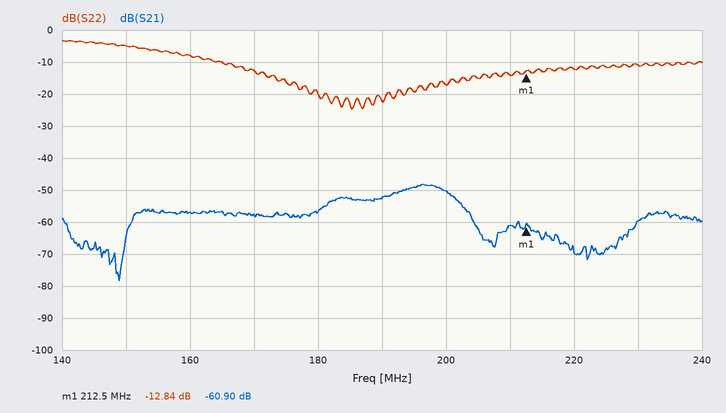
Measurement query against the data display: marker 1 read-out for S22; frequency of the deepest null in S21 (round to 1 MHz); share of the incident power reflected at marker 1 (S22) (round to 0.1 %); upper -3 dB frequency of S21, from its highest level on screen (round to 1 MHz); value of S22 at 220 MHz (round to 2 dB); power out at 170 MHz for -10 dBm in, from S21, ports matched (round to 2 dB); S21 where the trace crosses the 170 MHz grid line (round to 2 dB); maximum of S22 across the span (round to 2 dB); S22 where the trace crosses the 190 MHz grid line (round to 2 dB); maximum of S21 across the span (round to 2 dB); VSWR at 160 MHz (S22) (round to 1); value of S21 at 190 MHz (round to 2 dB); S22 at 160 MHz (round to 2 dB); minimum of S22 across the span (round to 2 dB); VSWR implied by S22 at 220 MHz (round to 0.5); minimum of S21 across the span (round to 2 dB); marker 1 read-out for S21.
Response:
-12.84 dB
149 MHz
5.2 %
201 MHz
-12 dB
-68 dBm
-58 dB
-4 dB
-22 dB
-48 dB
2
-52 dB
-8 dB
-24 dB
1.5
-78 dB
-60.90 dB
